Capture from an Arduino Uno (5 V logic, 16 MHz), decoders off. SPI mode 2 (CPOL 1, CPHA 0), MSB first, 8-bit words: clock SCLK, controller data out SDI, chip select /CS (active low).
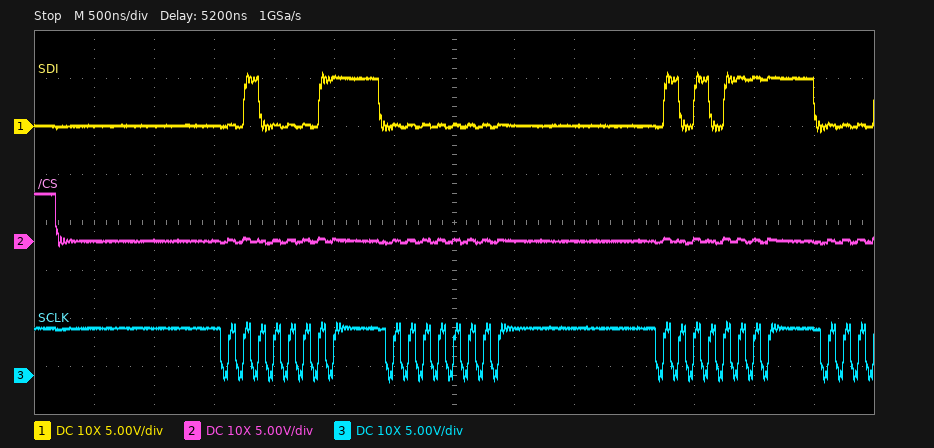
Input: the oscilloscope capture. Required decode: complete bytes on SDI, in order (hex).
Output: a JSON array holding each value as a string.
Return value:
["0x21 0x00 0x57"]
